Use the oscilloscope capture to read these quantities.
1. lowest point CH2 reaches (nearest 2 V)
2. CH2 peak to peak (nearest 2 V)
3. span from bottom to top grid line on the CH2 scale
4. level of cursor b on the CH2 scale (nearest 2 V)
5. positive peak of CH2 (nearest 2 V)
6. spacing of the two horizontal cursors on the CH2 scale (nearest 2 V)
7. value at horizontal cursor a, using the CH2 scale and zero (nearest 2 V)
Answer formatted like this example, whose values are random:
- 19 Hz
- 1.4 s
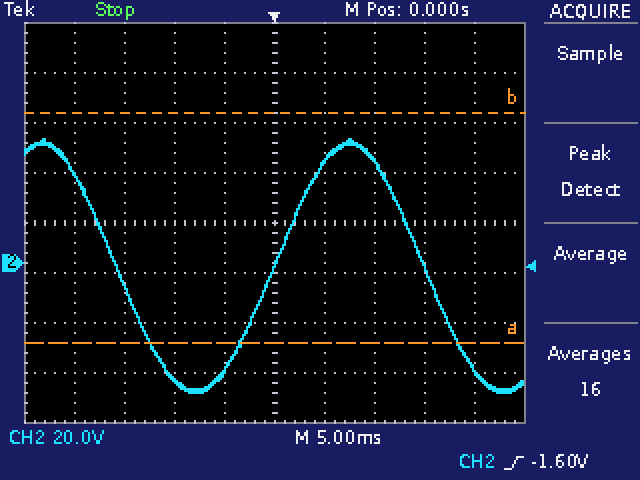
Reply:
- -52 V
- 102 V
- 160 V
- 60 V
- 50 V
- 92 V
- -32 V
